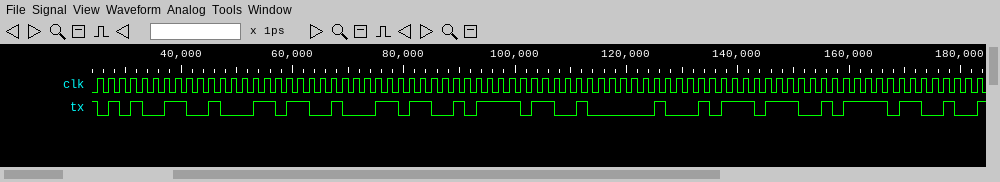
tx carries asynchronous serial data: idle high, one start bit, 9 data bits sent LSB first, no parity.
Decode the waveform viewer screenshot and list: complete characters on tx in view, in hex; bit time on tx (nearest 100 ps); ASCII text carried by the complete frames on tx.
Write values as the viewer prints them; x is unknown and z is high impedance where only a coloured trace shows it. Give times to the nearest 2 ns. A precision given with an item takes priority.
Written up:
65, 6C, 6C, 6F, 20, 77, 6F
2000 ps
"ello wo"
